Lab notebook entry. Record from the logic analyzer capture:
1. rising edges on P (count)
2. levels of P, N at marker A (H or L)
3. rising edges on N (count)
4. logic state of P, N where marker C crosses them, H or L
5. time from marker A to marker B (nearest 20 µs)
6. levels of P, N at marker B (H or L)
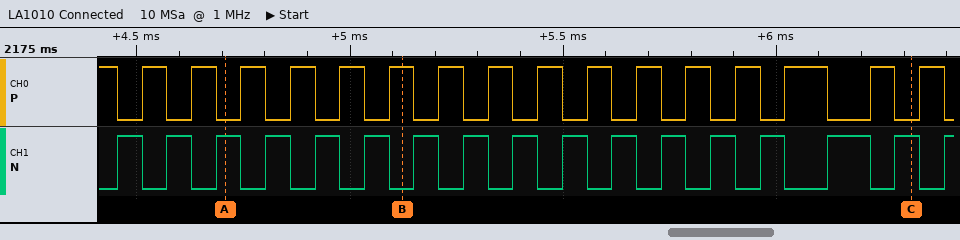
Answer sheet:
16
P=L, N=H
17
P=L, N=H
420 µs
P=H, N=L
